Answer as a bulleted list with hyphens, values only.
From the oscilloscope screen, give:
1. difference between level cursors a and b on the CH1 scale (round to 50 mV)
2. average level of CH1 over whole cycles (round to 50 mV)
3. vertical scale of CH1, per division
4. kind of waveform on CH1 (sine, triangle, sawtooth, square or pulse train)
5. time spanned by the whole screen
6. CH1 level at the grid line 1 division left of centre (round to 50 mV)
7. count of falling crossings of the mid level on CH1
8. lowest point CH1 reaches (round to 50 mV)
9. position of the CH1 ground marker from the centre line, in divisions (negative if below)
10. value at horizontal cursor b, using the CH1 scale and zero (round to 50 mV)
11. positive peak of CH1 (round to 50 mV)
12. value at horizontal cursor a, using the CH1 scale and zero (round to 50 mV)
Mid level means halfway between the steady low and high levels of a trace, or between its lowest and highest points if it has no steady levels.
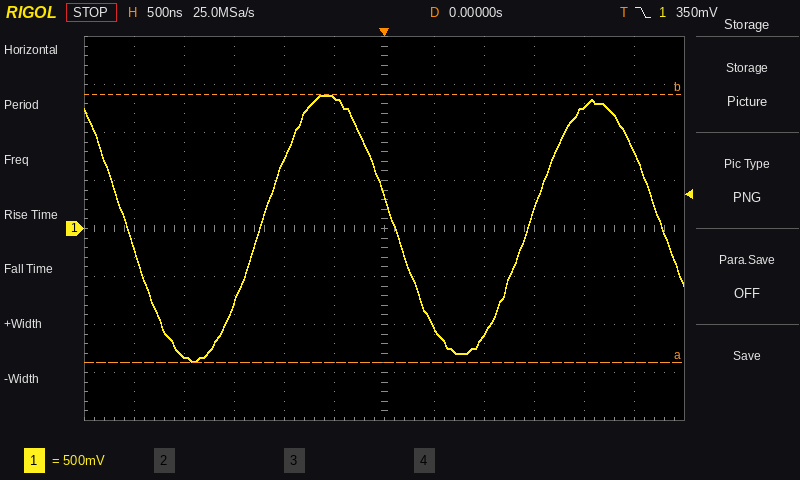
- 2.80 V
- 0 mV
- 500 mV
- sine
- 6 µs
- 1.35 V
- 3
- -1.40 V
- 0.0 div
- 1.40 V
- 1.40 V
- -1.40 V
